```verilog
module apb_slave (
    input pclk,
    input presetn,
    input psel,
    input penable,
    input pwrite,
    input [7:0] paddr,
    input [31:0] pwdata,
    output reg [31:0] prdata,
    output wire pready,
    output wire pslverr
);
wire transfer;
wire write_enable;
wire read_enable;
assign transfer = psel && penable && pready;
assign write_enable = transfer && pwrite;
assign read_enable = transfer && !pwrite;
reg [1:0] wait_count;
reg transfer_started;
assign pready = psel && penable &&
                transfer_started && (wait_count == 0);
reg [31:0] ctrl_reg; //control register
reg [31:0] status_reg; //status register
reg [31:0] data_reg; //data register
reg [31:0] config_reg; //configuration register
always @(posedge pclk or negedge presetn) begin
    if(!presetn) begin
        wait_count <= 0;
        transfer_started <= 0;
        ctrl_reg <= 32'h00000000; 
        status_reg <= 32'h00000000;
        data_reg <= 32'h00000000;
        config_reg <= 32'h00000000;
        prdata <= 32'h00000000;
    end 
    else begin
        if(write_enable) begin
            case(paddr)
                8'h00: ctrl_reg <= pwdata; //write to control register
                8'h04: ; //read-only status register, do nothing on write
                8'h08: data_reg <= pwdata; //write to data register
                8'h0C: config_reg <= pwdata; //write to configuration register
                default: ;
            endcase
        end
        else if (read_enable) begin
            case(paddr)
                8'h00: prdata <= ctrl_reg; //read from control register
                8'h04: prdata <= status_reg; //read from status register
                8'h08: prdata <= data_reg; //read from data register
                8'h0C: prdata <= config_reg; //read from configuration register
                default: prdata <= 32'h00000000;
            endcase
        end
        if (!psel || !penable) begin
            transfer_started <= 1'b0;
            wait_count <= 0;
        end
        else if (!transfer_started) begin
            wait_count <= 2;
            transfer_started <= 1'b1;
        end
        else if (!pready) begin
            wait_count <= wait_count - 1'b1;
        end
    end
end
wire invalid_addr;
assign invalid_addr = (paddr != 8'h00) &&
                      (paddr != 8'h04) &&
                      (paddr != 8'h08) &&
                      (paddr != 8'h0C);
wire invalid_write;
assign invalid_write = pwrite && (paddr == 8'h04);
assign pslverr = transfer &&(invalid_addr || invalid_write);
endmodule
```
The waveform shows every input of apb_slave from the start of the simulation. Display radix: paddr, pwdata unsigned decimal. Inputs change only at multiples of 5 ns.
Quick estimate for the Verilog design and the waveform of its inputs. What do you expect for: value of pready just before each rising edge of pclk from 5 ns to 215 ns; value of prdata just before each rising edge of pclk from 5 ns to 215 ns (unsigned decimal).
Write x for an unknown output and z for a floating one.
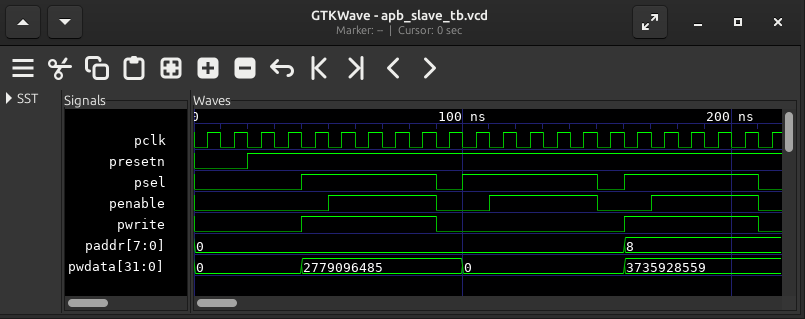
0 0 0 0 0 0 0 0 1 0 0 0 0 0 1 0 0 0 0 0 1 0
0, 0, 0, 0, 0, 0, 0, 0, 0, 0, 0, 0, 0, 0, 0, 2779096485, 2779096485, 2779096485, 2779096485, 2779096485, 2779096485, 2779096485
